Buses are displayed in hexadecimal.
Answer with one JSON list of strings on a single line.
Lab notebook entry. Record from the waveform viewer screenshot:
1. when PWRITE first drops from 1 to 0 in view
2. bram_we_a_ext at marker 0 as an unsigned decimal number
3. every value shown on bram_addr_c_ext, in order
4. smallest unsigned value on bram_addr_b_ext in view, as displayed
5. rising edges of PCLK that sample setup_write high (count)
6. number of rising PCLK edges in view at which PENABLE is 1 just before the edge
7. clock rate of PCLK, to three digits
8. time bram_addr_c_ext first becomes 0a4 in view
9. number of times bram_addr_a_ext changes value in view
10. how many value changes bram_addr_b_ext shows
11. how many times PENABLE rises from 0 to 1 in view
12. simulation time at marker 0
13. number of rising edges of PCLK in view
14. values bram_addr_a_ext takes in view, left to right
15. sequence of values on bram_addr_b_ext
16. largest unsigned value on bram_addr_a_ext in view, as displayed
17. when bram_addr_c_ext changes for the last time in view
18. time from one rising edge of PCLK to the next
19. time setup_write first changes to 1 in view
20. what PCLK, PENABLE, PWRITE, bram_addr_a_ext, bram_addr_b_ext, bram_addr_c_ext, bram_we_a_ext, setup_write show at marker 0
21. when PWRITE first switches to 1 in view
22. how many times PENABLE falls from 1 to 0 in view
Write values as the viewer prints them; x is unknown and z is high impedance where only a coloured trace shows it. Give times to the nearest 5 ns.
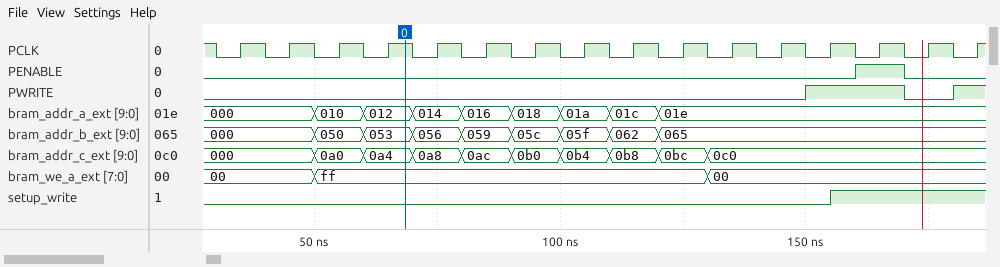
["170 ns", "255", "000, 0a0, 0a4, 0a8, 0ac, 0b0, 0b4, 0b8, 0bc, 0c0", "000", "3", "1", "100 MHz", "60 ns", "8", "8", "1", "70 ns", "16", "000, 010, 012, 014, 016, 018, 01a, 01c, 01e", "000, 050, 053, 056, 059, 05c, 05f, 062, 065", "01e", "130 ns", "10 ns", "155 ns", "PCLK=1, PENABLE=0, PWRITE=0, bram_addr_a_ext=012, bram_addr_b_ext=053, bram_addr_c_ext=0a4, bram_we_a_ext=ff, setup_write=0", "150 ns", "1"]
